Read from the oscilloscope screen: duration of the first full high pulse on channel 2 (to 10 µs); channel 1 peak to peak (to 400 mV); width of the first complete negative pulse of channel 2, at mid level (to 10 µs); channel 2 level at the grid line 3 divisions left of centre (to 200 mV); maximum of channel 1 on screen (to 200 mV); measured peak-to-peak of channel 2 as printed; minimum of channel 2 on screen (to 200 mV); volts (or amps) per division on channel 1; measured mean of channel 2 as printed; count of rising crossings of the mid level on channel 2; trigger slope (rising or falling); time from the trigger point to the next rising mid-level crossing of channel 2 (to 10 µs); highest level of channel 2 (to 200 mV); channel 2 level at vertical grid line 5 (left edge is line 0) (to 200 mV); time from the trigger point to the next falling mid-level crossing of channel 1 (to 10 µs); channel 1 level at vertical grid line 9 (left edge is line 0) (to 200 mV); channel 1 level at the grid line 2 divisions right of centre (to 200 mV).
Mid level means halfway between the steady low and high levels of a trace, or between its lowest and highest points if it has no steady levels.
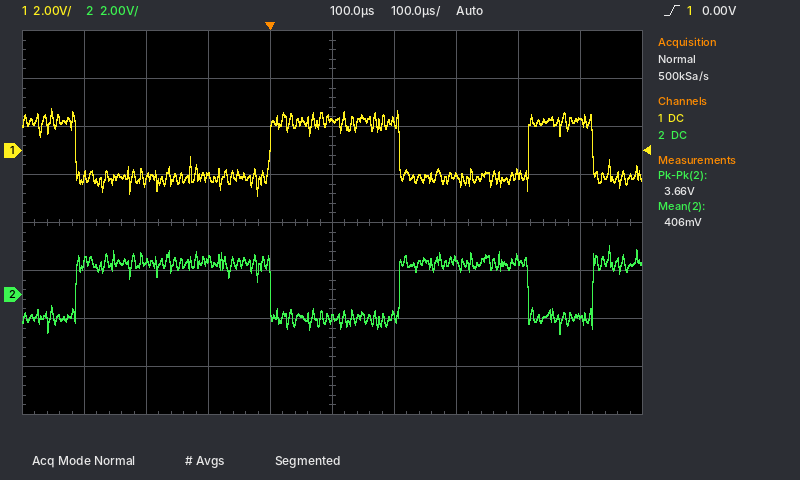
310 µs
3.6 V
210 µs
1.4 V
1.8 V
3.66 V
-1.6 V
2 V
406 mV
3
rising
210 µs
2.0 V
-1.0 V
210 µs
1.2 V
-1.0 V
